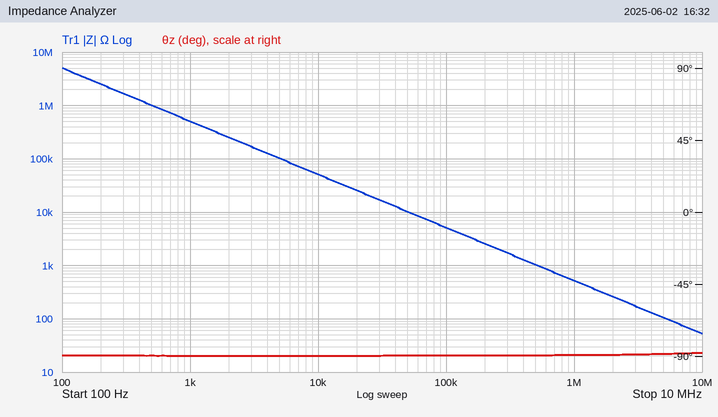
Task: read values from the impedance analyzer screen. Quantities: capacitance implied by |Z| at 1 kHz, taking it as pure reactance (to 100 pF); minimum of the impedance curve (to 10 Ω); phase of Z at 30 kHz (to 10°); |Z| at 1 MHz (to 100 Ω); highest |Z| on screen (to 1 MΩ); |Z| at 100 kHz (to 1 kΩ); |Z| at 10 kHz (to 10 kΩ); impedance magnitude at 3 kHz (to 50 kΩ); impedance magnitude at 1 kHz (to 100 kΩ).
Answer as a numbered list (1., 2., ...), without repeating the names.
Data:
1. 300 pF
2. 50 Ω
3. -90°
4. 500 Ω
5. 5 MΩ
6. 5 kΩ
7. 50 kΩ
8. 150 kΩ
9. 500 kΩ
